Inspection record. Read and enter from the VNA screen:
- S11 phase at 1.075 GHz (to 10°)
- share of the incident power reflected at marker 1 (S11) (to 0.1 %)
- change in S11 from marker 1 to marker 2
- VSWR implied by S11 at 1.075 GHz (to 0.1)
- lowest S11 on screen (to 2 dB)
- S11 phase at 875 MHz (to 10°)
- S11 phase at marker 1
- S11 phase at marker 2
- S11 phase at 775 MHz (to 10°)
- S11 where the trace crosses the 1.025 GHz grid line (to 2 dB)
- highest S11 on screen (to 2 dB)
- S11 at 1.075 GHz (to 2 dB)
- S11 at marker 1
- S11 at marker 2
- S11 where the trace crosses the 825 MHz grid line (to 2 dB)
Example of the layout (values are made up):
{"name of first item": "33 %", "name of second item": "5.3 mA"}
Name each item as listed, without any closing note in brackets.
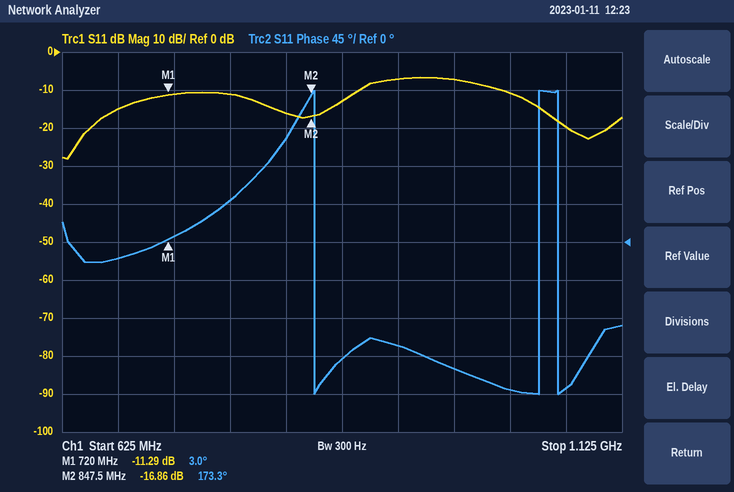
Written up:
{"S11 phase at 1.075 GHz": "-170°", "share of the incident power reflected at marker 1 (S11)": "7.4 %", "change in S11 from marker 1 to marker 2": "-5.57 dB", "VSWR implied by S11 at 1.075 GHz": "1.2", "lowest S11 on screen": "-28 dB", "S11 phase at 875 MHz": "-140°", "S11 phase at marker 1": "3.0°", "S11 phase at marker 2": "173.3°", "S11 phase at 775 MHz": "50°", "S11 where the trace crosses the 1.025 GHz grid line": "-10 dB", "highest S11 on screen": "-6 dB", "S11 at 1.075 GHz": "-20 dB", "S11 at marker 1": "-11.29 dB", "S11 at marker 2": "-16.86 dB", "S11 where the trace crosses the 825 MHz grid line": "-16 dB"}
